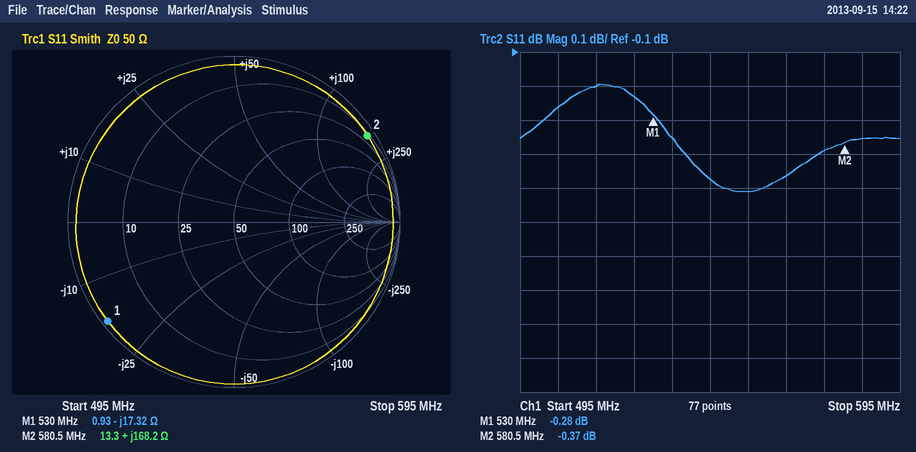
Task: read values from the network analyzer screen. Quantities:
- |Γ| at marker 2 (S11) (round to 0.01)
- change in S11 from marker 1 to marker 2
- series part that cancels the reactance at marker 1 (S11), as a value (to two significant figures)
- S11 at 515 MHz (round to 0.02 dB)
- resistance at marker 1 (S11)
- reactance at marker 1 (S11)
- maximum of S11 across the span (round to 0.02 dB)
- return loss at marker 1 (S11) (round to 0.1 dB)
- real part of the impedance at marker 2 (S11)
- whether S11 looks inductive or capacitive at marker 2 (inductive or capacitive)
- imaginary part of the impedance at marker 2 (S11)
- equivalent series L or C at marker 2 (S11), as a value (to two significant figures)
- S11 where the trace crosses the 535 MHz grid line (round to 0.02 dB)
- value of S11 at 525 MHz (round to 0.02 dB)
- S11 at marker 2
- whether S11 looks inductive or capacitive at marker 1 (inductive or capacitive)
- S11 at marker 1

0.96
-0.09 dB
5.2 nH
-0.20 dB
0.93 Ω
-17.32 Ω
-0.20 dB
0.3 dB
13.3 Ω
inductive
+168.2 Ω
46 nH
-0.36 dB
-0.24 dB
-0.37 dB
capacitive
-0.28 dB
